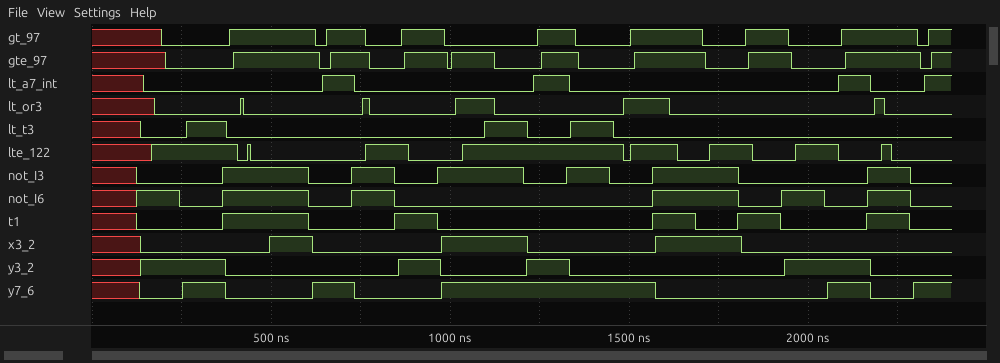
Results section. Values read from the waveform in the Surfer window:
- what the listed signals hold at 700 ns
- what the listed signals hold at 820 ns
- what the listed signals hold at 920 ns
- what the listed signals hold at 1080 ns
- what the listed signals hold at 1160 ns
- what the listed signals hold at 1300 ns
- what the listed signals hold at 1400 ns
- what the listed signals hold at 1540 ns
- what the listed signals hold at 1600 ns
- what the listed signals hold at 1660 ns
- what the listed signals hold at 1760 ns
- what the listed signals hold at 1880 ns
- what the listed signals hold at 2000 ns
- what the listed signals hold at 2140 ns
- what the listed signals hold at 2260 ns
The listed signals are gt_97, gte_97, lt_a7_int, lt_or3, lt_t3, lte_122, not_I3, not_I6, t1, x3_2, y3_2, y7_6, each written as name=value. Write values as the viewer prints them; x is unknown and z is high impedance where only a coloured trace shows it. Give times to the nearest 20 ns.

gt_97=1, gte_97=1, lt_a7_int=1, lt_or3=0, lt_t3=0, lte_122=0, not_I3=0, not_I6=0, t1=0, x3_2=0, y3_2=0, y7_6=1
gt_97=0, gte_97=0, lt_a7_int=0, lt_or3=0, lt_t3=0, lte_122=1, not_I3=1, not_I6=1, t1=0, x3_2=0, y3_2=0, y7_6=0
gt_97=1, gte_97=1, lt_a7_int=0, lt_or3=0, lt_t3=0, lte_122=0, not_I3=0, not_I6=0, t1=1, x3_2=0, y3_2=1, y7_6=0
gt_97=0, gte_97=1, lt_a7_int=0, lt_or3=1, lt_t3=0, lte_122=1, not_I3=1, not_I6=0, t1=0, x3_2=1, y3_2=0, y7_6=1
gt_97=0, gte_97=0, lt_a7_int=0, lt_or3=0, lt_t3=1, lte_122=1, not_I3=1, not_I6=0, t1=0, x3_2=1, y3_2=0, y7_6=1
gt_97=1, gte_97=1, lt_a7_int=1, lt_or3=0, lt_t3=0, lte_122=1, not_I3=0, not_I6=0, t1=0, x3_2=0, y3_2=1, y7_6=1
gt_97=0, gte_97=0, lt_a7_int=0, lt_or3=0, lt_t3=1, lte_122=1, not_I3=1, not_I6=0, t1=0, x3_2=0, y3_2=0, y7_6=1
gt_97=1, gte_97=1, lt_a7_int=0, lt_or3=1, lt_t3=0, lte_122=1, not_I3=0, not_I6=0, t1=0, x3_2=0, y3_2=0, y7_6=1
gt_97=1, gte_97=1, lt_a7_int=0, lt_or3=1, lt_t3=0, lte_122=1, not_I3=1, not_I6=1, t1=1, x3_2=1, y3_2=0, y7_6=0
gt_97=1, gte_97=1, lt_a7_int=0, lt_or3=0, lt_t3=0, lte_122=0, not_I3=1, not_I6=1, t1=1, x3_2=1, y3_2=0, y7_6=0
gt_97=0, gte_97=0, lt_a7_int=0, lt_or3=0, lt_t3=0, lte_122=1, not_I3=1, not_I6=1, t1=0, x3_2=1, y3_2=0, y7_6=0
gt_97=1, gte_97=1, lt_a7_int=0, lt_or3=0, lt_t3=0, lte_122=0, not_I3=0, not_I6=0, t1=1, x3_2=0, y3_2=0, y7_6=0
gt_97=0, gte_97=0, lt_a7_int=0, lt_or3=0, lt_t3=0, lte_122=1, not_I3=0, not_I6=1, t1=0, x3_2=0, y3_2=1, y7_6=0
gt_97=1, gte_97=1, lt_a7_int=1, lt_or3=0, lt_t3=0, lte_122=0, not_I3=0, not_I6=0, t1=0, x3_2=0, y3_2=1, y7_6=1
gt_97=1, gte_97=1, lt_a7_int=0, lt_or3=0, lt_t3=0, lte_122=0, not_I3=1, not_I6=1, t1=1, x3_2=0, y3_2=0, y7_6=0
